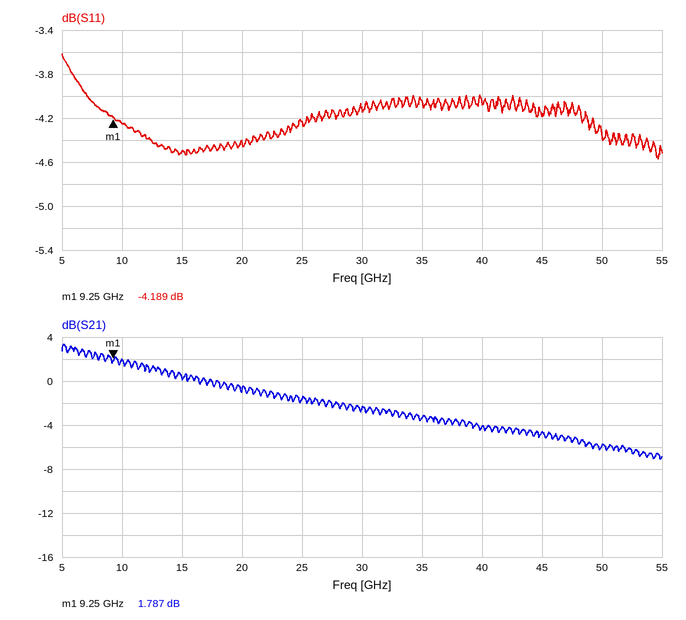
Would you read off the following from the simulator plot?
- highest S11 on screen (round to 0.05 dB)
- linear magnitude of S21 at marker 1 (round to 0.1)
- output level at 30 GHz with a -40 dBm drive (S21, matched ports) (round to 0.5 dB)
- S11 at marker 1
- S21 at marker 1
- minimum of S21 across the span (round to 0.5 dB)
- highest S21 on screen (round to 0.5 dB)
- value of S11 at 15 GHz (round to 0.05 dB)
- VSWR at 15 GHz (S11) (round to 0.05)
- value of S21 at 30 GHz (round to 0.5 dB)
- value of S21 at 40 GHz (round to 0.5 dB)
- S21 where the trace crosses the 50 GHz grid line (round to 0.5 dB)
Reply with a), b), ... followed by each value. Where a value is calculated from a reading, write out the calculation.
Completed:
a) -3.60 dB
b) 10^(1.787/20) ≈ 1.2
c) -40 dBm + (-2.5 dB) = -42.5 dBm
d) -4.189 dB
e) 1.787 dB
f) -7.0 dB
g) 3.5 dB
h) -4.50 dB
i) |Γ| = 10^(-4.5/20) = 0.5957; VSWR = (1 + 0.5957)/(1 − 0.5957) ≈ 3.95
j) -2.5 dB
k) -4.0 dB
l) -6.0 dB
